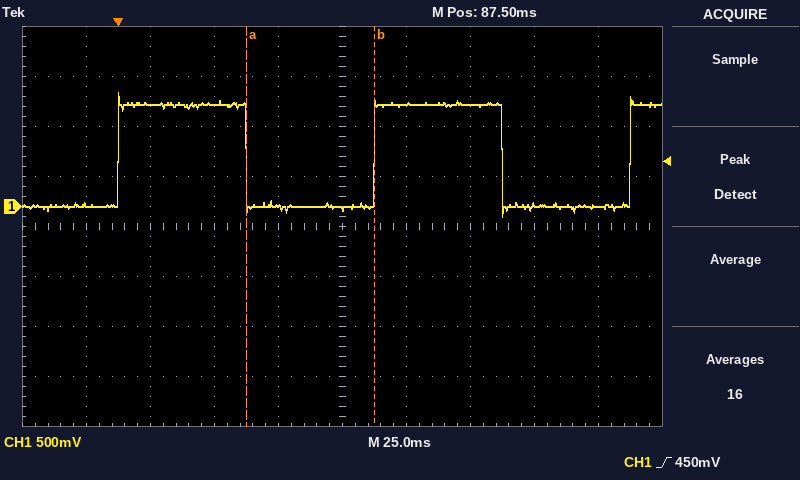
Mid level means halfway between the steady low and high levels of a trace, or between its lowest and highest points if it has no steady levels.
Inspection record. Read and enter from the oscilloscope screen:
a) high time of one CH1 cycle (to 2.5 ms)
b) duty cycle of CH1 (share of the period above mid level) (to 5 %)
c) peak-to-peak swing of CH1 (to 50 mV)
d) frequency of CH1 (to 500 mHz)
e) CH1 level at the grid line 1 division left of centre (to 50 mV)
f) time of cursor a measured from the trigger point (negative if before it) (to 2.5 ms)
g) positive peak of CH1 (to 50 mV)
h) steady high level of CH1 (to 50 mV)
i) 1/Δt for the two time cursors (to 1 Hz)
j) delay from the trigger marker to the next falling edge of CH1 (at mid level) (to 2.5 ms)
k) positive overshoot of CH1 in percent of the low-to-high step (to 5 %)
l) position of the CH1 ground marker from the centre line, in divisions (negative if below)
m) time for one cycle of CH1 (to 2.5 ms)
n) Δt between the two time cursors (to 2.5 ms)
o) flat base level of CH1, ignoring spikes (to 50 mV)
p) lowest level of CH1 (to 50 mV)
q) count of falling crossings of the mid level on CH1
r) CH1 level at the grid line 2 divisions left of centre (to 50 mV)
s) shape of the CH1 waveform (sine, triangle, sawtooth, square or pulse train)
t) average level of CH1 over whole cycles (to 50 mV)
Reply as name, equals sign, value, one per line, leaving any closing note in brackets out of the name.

high time of one CH1 cycle = 50.0 ms
duty cycle of CH1 (share of the period above mid level) = 50 %
peak-to-peak swing of CH1 = 1.25 V
frequency of CH1 = 10.0 Hz
CH1 level at the grid line 1 division left of centre = 0 mV
time of cursor a measured from the trigger point (negative if before it) = +50.0 ms
positive peak of CH1 = 1.15 V
steady high level of CH1 = 1.00 V
1/Δt for the two time cursors = 20 Hz
delay from the trigger marker to the next falling edge of CH1 (at mid level) = 50.0 ms
positive overshoot of CH1 in percent of the low-to-high step = 10 %
position of the CH1 ground marker from the centre line, in divisions = +0.4 div
time for one cycle of CH1 = 100.0 ms
Δt between the two time cursors = 50.0 ms
flat base level of CH1, ignoring spikes = 0 mV
lowest level of CH1 = -100 mV
count of falling crossings of the mid level on CH1 = 2
CH1 level at the grid line 2 divisions left of centre = 1.00 V
shape of the CH1 waveform = square
average level of CH1 over whole cycles = 500 mV
